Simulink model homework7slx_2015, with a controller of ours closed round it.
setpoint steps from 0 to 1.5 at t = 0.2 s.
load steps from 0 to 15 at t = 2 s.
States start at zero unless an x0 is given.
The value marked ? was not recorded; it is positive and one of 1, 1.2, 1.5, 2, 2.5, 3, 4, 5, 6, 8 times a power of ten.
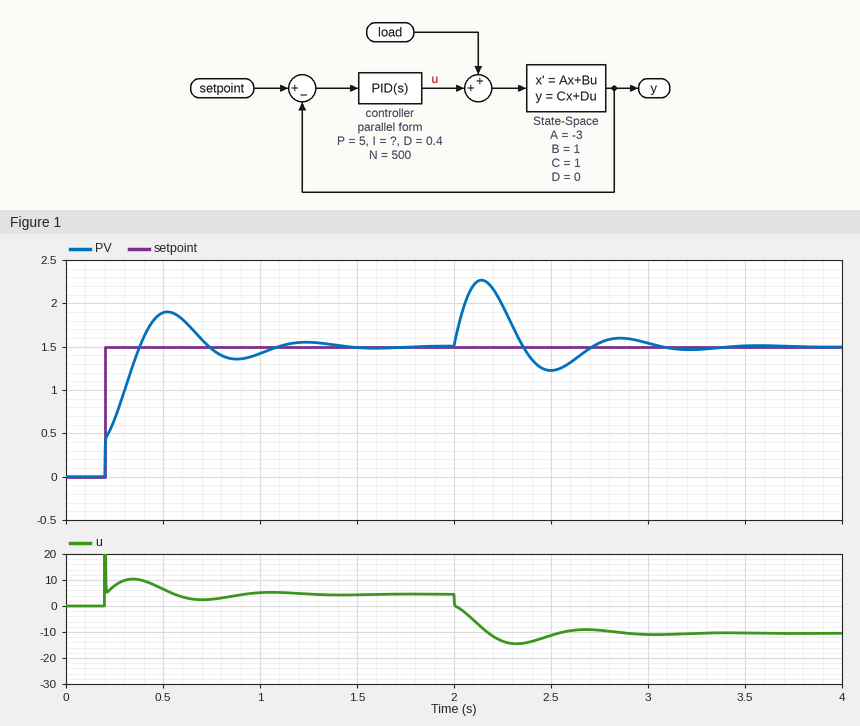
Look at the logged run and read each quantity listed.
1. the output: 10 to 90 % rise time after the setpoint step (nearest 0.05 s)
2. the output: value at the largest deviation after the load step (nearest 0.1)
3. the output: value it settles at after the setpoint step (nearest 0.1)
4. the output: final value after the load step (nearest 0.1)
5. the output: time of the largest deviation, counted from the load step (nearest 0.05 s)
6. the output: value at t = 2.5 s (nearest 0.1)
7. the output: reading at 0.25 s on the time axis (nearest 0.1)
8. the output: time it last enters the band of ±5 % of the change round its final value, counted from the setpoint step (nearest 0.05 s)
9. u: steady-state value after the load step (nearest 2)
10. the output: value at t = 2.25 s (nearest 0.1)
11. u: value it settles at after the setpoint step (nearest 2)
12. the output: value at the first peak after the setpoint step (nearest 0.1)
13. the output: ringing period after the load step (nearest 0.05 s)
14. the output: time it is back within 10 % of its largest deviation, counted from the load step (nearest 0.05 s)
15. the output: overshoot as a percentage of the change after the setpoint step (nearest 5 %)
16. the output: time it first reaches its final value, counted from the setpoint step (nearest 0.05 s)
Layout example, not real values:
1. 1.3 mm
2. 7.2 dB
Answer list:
1. 0.15 s
2. 2.3
3. 1.5
4. 1.5
5. 0.15 s
6. 1.2
7. 0.7
8. 0.80 s
9. -10
10. 2.0
11. 4
12. 1.9
13. 0.70 s
14. 0.95 s
15. 25 %
16. 0.20 s
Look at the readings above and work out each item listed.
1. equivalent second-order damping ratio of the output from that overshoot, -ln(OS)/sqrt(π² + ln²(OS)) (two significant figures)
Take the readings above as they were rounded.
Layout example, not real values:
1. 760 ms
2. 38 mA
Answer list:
1. 0.40
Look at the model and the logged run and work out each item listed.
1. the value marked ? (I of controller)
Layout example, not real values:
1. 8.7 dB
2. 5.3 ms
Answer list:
1. 120
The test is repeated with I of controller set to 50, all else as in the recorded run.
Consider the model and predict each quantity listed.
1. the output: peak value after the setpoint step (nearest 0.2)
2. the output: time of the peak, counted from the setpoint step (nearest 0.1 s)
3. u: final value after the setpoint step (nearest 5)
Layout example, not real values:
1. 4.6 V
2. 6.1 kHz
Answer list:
1. 1.8
2. 0.5 s
3. 5
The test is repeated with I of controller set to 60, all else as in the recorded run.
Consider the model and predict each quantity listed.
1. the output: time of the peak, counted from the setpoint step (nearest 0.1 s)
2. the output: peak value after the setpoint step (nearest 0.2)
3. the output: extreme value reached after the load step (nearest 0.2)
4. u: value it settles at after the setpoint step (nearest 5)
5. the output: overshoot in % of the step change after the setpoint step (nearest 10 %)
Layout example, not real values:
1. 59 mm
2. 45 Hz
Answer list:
1. 0.5 s
2. 1.8
3. 2.4
4. 5
5. 20 %
